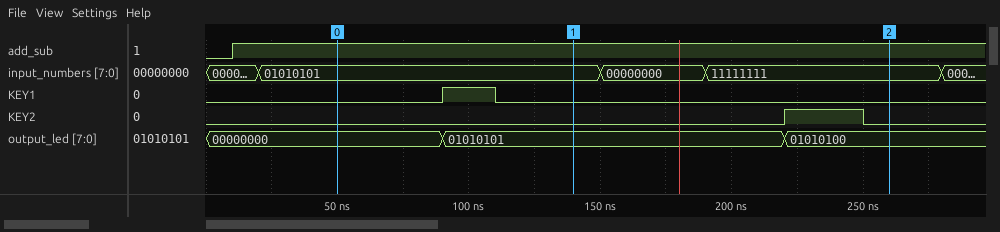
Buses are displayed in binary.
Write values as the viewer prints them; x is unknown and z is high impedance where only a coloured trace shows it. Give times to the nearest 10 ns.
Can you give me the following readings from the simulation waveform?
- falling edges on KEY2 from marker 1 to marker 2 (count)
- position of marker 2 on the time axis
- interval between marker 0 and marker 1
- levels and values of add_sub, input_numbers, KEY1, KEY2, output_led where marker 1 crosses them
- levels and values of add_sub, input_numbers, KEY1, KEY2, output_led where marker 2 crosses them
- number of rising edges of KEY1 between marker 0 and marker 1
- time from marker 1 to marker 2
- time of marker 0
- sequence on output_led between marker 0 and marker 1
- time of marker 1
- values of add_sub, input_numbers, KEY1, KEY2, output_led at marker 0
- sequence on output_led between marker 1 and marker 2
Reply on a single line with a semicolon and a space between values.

1; 260 ns; 90 ns; add_sub=1, input_numbers=01010101, KEY1=0, KEY2=0, output_led=01010101; add_sub=1, input_numbers=11111111, KEY1=0, KEY2=0, output_led=01010100; 1; 120 ns; 50 ns; 00000000, 01010101; 140 ns; add_sub=1, input_numbers=01010101, KEY1=0, KEY2=0, output_led=00000000; 01010101, 01010100
